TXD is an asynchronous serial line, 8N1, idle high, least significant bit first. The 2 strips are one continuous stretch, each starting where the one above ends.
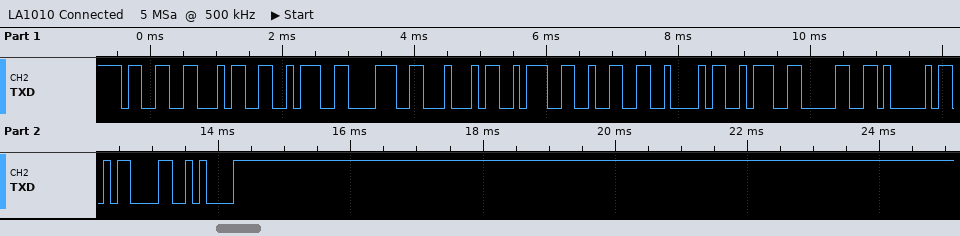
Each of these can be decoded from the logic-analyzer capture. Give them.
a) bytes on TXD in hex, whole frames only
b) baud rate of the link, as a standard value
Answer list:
0x33 0x34 0x3A 0x38 0x44 0x3A 0x32 0x42 0x3A 0x30 0x41 0x0D 0x0A
9600 baud
